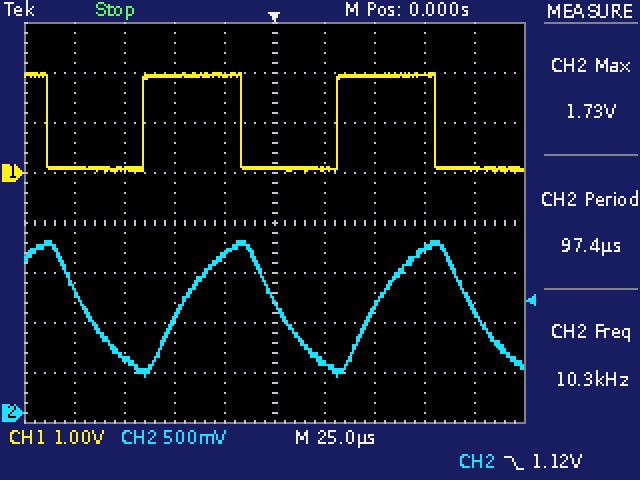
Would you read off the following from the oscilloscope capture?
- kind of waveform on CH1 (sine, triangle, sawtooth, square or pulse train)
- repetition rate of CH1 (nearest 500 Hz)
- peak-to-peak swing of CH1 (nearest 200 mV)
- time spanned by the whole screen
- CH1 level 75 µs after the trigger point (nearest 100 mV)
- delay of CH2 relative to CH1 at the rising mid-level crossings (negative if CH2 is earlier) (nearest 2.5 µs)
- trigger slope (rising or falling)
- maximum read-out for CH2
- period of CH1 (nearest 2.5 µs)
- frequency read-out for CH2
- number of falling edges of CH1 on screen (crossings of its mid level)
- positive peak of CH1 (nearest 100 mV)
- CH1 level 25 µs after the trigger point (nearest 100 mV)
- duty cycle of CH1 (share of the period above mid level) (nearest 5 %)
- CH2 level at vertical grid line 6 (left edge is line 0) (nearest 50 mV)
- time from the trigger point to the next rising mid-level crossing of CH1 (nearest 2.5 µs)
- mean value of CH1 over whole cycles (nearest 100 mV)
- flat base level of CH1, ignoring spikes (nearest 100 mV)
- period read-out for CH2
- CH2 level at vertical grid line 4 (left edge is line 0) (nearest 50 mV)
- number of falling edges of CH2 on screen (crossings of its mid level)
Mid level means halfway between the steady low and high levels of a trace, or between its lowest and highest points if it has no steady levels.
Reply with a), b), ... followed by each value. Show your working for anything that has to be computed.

a) square
b) 1 / 97.5 µs ≈ 10.3 kHz, so 10.5 kHz to the nearest 500 Hz
c) 2.0 V
d) 250 µs
e) 2.0 V
f) +17.5 µs
g) falling
h) 1.73 V
i) 97.5 µs
j) 10.3 kHz
k) 3
l) 2.0 V
m) 100 mV
n) 50 %
o) 500 mV
p) 32.5 µs
q) 100 mV + 0.5 × (2.0 V − (100 mV)) ≈ 1.0 V
r) 100 mV
s) 97.4 µs
t) 1.60 V
u) 3
